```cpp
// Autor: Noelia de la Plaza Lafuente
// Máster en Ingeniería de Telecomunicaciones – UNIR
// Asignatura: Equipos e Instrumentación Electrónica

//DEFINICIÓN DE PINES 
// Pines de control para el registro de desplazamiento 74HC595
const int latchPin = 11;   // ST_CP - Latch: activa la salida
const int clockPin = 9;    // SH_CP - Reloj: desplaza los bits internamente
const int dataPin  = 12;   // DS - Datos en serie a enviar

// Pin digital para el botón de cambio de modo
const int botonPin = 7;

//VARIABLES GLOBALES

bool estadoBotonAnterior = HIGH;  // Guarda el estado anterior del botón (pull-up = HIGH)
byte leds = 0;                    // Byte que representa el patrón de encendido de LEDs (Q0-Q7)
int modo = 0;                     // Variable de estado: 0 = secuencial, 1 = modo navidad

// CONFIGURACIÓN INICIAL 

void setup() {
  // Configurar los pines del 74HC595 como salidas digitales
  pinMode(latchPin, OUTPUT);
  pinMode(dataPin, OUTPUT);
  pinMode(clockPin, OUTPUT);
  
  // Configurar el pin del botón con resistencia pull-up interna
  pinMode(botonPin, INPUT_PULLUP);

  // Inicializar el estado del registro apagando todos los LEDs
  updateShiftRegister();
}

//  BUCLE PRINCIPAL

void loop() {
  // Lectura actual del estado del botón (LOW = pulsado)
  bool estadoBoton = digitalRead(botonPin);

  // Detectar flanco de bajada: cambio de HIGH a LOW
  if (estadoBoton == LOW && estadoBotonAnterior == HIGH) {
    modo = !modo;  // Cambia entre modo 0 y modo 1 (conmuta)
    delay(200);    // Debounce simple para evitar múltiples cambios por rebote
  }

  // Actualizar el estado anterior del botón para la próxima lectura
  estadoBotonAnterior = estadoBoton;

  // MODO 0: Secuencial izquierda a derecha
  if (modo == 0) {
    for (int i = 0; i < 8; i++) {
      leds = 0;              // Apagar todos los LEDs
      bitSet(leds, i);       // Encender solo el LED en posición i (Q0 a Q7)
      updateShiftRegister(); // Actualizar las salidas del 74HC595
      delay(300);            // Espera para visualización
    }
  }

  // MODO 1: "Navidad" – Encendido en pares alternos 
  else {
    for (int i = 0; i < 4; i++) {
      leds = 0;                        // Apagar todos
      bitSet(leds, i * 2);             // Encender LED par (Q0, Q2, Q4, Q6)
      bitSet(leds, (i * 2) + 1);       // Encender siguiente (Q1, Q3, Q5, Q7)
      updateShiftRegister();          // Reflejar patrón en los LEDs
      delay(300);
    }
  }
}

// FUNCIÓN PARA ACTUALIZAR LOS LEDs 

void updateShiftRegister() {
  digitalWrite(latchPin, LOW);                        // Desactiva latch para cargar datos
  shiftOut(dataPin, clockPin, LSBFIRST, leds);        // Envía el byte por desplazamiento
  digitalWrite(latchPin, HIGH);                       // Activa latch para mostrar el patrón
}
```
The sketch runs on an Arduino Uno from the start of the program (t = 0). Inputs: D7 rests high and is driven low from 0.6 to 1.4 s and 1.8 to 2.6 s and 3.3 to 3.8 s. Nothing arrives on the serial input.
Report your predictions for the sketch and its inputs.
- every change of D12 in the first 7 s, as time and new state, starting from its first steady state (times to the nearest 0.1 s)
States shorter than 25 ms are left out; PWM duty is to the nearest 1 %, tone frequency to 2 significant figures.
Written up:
0 s low; 2.1 s high; 2.6 s low; 3.5 s high; 3.8 s low; 4.7 s high; 5 s low; 5.9 s high; 6.2 s low
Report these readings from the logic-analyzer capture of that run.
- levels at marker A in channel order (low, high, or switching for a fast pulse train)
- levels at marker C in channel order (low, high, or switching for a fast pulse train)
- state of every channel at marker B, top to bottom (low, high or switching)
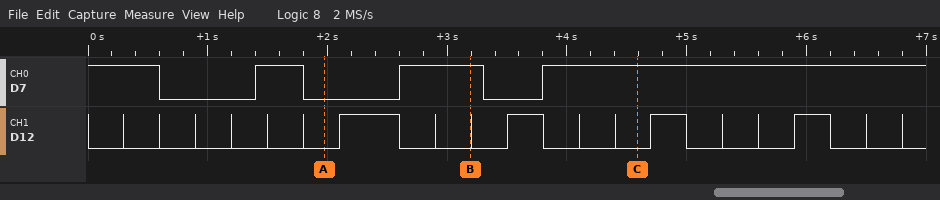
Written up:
D7 low, D12 low
D7 high, D12 low
D7 high, D12 low
